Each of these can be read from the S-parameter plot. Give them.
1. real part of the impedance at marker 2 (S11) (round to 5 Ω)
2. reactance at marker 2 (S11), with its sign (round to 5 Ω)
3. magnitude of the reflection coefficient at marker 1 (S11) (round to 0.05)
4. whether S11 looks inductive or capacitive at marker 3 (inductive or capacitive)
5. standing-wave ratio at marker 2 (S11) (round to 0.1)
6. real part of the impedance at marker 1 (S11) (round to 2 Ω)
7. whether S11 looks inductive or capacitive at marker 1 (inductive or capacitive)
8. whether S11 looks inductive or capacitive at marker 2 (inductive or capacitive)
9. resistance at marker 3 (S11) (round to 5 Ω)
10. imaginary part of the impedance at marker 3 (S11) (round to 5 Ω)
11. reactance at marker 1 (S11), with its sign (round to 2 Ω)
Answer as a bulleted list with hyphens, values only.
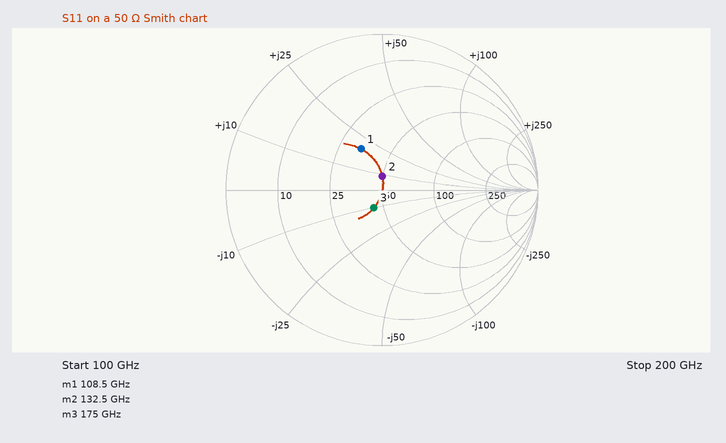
- 50 Ω
- +10 Ω
- 0.30
- capacitive
- 1.2
- 34 Ω
- inductive
- inductive
- 45 Ω
- -10 Ω
- +20 Ω
